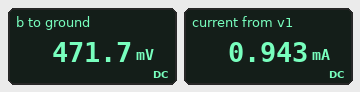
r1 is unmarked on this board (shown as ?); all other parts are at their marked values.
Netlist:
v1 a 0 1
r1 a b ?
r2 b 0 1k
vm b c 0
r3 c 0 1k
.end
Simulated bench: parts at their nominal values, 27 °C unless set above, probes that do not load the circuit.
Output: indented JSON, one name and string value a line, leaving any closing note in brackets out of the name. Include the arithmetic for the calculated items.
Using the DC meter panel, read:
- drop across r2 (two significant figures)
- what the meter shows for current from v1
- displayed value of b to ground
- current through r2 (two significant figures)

{
  "drop across r2": "471.7 mV = 470 mV",
  "what the meter shows for current from v1": "0.943 mA",
  "displayed value of b to ground": "471.7 mV",
  "current through r2": "(471.7 mV) / 1 kΩ = 470 µA"
}
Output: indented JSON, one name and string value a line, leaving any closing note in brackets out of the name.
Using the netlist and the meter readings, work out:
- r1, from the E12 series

{
  "r1, from the E12 series": "560 Ω"
}
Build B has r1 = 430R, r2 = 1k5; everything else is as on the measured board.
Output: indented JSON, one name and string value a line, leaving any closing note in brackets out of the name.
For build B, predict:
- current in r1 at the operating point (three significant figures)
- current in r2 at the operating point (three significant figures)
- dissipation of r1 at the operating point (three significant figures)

{
  "current in r1 at the operating point": "971 µA",
  "current in r2 at the operating point": "388 µA",
  "dissipation of r1 at the operating point": "405 µW"
}
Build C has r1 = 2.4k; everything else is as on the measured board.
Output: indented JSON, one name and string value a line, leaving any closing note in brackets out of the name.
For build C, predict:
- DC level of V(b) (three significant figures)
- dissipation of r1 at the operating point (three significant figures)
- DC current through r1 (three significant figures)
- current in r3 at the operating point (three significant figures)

{
  "DC level of V(b)": "172 mV",
  "dissipation of r1 at the operating point": "285 µW",
  "DC current through r1": "345 µA",
  "current in r3 at the operating point": "172 µA"
}
